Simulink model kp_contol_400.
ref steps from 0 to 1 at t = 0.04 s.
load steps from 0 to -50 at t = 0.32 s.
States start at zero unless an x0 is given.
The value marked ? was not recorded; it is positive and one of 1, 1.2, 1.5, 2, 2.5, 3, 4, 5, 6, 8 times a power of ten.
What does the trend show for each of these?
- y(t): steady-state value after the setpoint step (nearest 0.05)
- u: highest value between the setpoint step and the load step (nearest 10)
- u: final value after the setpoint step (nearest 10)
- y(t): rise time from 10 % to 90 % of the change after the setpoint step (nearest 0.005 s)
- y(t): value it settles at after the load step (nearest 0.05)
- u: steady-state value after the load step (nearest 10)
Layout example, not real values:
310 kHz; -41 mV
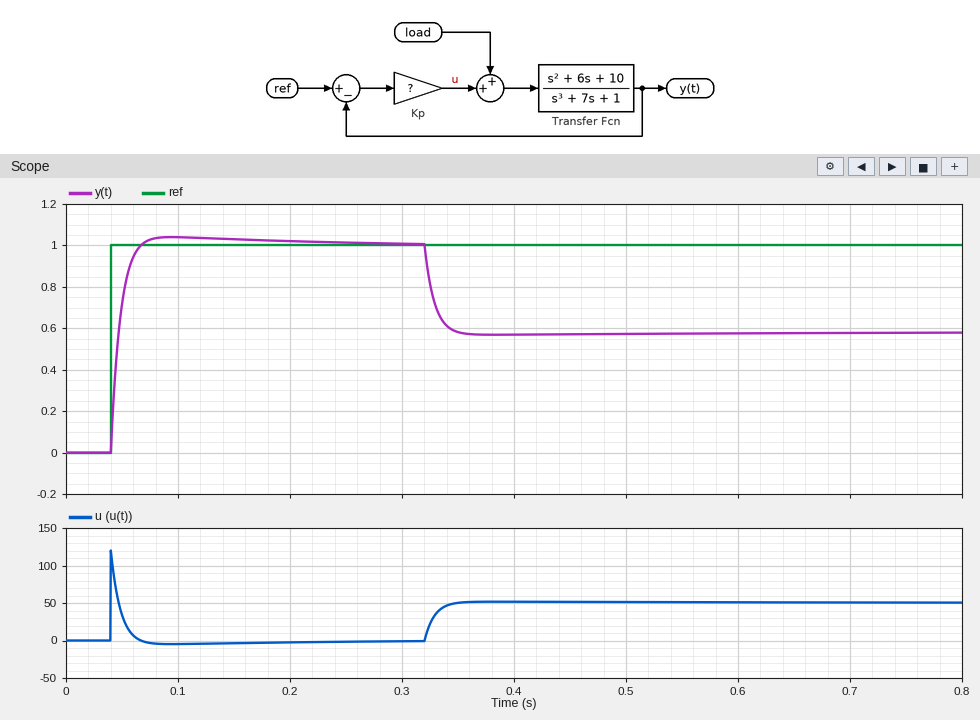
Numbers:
1.00; 120; 0; 0.015 s; 0.60; 50
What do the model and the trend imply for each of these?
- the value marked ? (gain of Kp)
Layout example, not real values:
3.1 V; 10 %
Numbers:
120
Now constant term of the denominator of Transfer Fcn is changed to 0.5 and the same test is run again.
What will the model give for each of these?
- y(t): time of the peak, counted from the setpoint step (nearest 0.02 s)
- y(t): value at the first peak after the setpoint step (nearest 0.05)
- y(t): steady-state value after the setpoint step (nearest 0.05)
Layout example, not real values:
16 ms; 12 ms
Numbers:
0.06 s; 1.05; 1.00
